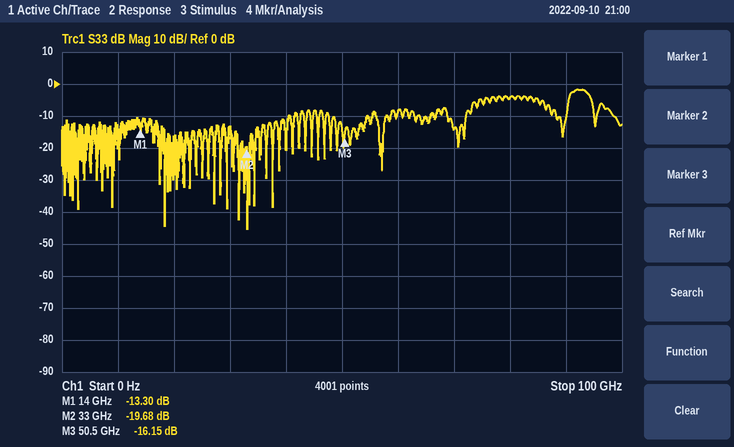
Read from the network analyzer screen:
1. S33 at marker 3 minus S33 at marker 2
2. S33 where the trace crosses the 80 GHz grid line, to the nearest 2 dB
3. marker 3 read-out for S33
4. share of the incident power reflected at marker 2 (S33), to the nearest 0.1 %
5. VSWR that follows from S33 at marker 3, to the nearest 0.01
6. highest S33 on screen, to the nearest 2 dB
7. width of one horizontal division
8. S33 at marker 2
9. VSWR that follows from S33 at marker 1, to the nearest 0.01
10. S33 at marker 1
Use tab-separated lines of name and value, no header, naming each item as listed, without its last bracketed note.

S33 at marker 3 minus S33 at marker 2	3.53 dB
S33 where the trace crosses the 80 GHz grid line, to the nearest 2 dB	-4 dB
marker 3 read-out for S33	-16.15 dB
share of the incident power reflected at marker 2 (S33), to the nearest 0.1 %	1.1 %
VSWR that follows from S33 at marker 3, to the nearest 0.01	1.37
highest S33 on screen, to the nearest 2 dB	-2 dB
width of one horizontal division	10 GHz
S33 at marker 2	-19.68 dB
VSWR that follows from S33 at marker 1, to the nearest 0.01	1.55
S33 at marker 1	-13.30 dB
